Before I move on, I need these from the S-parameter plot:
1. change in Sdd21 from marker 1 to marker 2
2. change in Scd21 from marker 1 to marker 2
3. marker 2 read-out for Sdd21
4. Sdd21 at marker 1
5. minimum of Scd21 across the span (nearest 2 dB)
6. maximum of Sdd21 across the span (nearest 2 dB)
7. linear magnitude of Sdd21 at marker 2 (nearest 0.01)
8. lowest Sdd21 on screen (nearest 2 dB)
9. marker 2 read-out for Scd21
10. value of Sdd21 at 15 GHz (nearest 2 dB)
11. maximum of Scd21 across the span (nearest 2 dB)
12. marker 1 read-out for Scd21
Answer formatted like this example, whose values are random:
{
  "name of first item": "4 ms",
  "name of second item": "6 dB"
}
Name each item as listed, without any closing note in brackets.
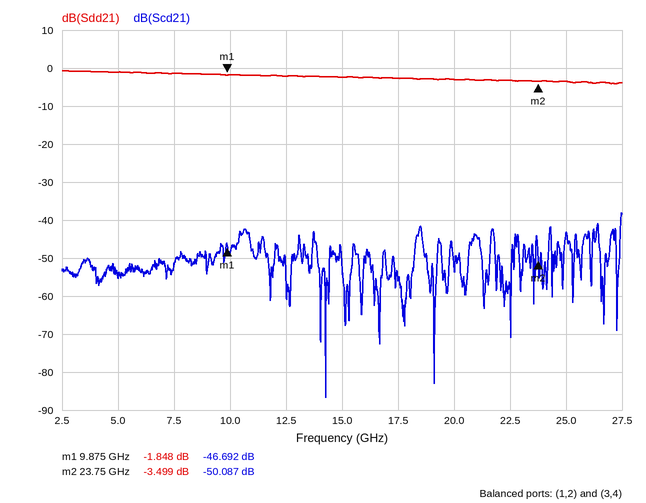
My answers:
{
  "change in Sdd21 from marker 1 to marker 2": "-1.651 dB",
  "change in Scd21 from marker 1 to marker 2": "-3.395 dB",
  "marker 2 read-out for Sdd21": "-3.499 dB",
  "Sdd21 at marker 1": "-1.848 dB",
  "minimum of Scd21 across the span": "-86 dB",
  "maximum of Sdd21 across the span": "0 dB",
  "linear magnitude of Sdd21 at marker 2": "0.67",
  "lowest Sdd21 on screen": "-4 dB",
  "marker 2 read-out for Scd21": "-50.087 dB",
  "value of Sdd21 at 15 GHz": "-2 dB",
  "maximum of Scd21 across the span": "-38 dB",
  "marker 1 read-out for Scd21": "-46.692 dB"
}
